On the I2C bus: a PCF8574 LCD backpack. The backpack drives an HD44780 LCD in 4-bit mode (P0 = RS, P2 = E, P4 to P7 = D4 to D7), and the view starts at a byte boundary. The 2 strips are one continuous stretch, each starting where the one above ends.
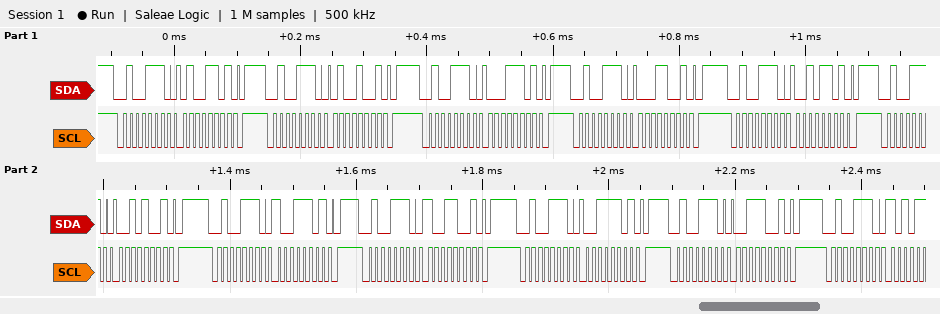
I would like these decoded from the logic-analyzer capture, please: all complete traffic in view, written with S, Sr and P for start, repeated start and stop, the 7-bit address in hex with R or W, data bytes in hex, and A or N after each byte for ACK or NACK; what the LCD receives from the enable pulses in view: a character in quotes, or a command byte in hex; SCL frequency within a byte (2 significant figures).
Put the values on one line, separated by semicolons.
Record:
S 27W A 4D A P S 27W A 49 A P S 27W A 1D A P S 27W A 19 A P S 27W A 2D A P S 27W A 29 A P S 27W A 9D A P S 27W A 99 A P S 27W A 3D A P S 27W A 39 A P S 27W A; 'A' ')'; 100 kHz
